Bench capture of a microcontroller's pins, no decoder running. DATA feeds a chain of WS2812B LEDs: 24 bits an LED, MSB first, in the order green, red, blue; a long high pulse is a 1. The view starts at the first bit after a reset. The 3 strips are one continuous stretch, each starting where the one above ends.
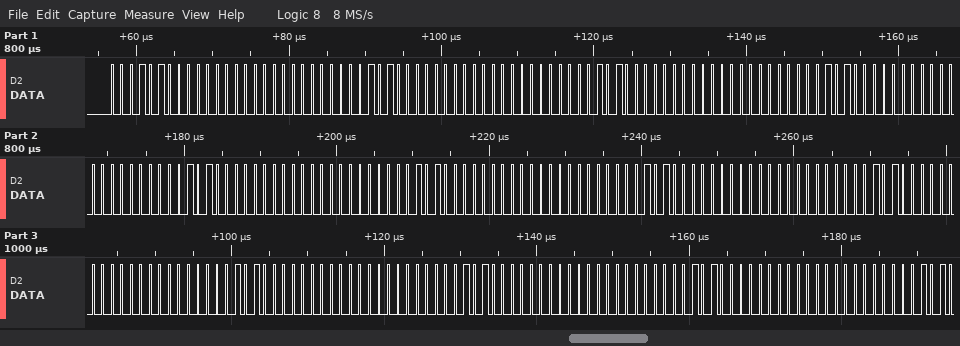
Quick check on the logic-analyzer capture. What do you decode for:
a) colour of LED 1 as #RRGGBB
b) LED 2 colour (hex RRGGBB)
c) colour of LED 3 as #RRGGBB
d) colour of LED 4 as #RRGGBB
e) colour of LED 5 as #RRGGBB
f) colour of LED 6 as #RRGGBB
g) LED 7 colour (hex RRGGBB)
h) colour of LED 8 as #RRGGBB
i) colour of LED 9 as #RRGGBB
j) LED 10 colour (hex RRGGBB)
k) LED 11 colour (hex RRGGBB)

#001400
#001400
#001400
#001400
#001400
#001400
#001400
#001400
#001400
#001400
#001400
